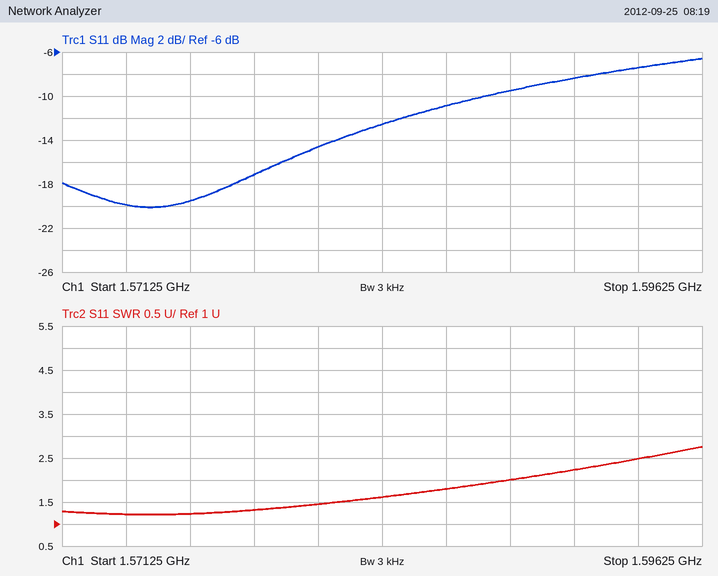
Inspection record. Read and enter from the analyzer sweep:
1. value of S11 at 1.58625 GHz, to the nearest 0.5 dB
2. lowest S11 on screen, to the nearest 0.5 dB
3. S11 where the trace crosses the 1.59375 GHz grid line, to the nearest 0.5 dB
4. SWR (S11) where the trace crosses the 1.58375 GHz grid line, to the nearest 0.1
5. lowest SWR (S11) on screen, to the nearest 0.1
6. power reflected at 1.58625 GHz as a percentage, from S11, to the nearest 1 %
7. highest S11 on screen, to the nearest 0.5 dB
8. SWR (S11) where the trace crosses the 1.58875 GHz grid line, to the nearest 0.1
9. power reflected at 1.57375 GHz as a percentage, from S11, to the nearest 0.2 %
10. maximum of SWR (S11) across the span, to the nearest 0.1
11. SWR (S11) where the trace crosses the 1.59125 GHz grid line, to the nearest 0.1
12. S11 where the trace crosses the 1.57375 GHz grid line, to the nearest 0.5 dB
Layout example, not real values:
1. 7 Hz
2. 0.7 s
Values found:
1. -11.0 dB
2. -20.0 dB
3. -7.5 dB
4. 1.6
5. 1.2
6. 8 %
7. -6.5 dB
8. 2.0
9. 1.0 %
10. 2.8
11. 2.2
12. -20.0 dB
